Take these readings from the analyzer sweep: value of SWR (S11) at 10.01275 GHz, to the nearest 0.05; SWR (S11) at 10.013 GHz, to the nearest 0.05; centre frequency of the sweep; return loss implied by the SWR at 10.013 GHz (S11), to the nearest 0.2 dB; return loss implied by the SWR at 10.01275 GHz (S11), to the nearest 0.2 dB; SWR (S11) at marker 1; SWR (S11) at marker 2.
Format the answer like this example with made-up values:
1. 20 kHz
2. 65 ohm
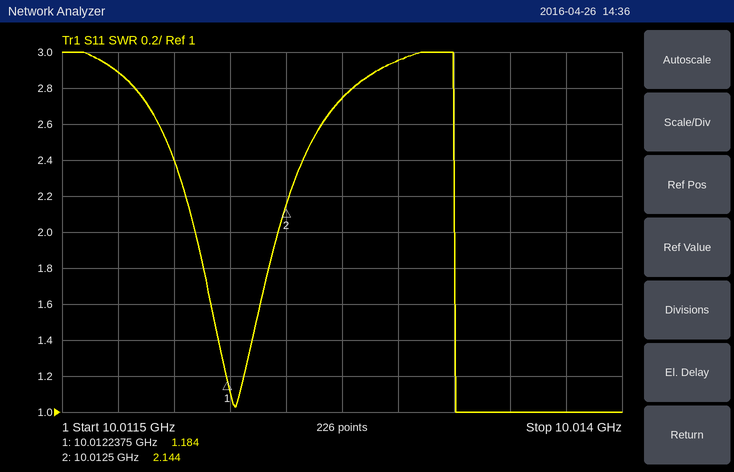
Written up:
1. 2.75
2. 2.95
3. 10.01275 GHz
4. 6.2 dB
5. 6.6 dB
6. 1.184
7. 2.144
